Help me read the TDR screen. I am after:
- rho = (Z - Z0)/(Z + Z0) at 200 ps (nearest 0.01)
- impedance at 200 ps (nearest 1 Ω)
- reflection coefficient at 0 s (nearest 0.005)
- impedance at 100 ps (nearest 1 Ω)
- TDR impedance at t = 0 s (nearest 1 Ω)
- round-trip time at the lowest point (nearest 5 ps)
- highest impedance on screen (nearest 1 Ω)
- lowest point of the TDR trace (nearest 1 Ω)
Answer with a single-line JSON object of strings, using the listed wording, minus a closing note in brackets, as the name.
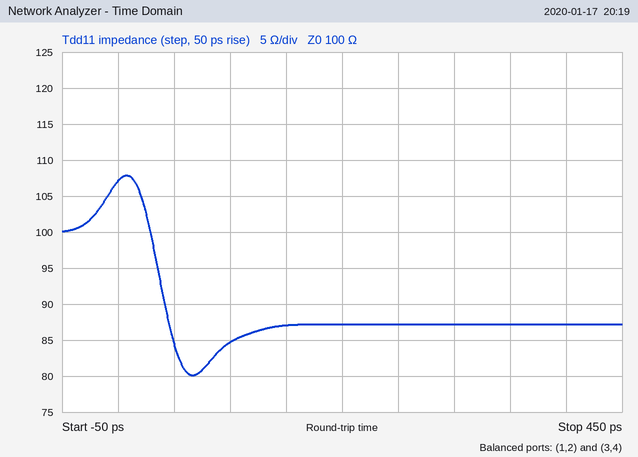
{"rho = (Z - Z0)/(Z + Z0) at 200 ps": "-0.07", "impedance at 200 ps": "87 Ω", "reflection coefficient at 0 s": "+0.035", "impedance at 100 ps": "85 Ω", "TDR impedance at t = 0 s": "107 Ω", "round-trip time at the lowest point": "65 ps", "highest impedance on screen": "108 Ω", "lowest point of the TDR trace": "80 Ω"}
